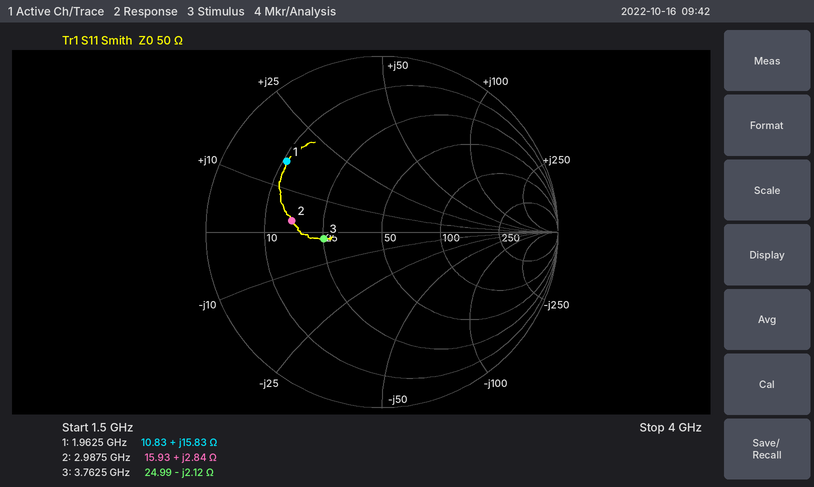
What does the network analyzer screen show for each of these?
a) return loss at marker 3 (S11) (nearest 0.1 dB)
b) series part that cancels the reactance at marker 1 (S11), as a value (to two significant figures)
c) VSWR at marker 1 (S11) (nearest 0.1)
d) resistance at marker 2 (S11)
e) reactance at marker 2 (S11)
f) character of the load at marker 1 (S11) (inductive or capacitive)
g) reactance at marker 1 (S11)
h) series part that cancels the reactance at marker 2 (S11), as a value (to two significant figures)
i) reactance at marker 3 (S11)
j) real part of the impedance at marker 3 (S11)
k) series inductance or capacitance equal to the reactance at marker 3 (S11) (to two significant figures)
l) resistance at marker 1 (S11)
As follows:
9.5 dB
5.1 pF
5.1
15.93 Ω
+2.84 Ω
inductive
+15.83 Ω
19 pF
-2.12 Ω
24.99 Ω
20 pF
10.83 Ω
